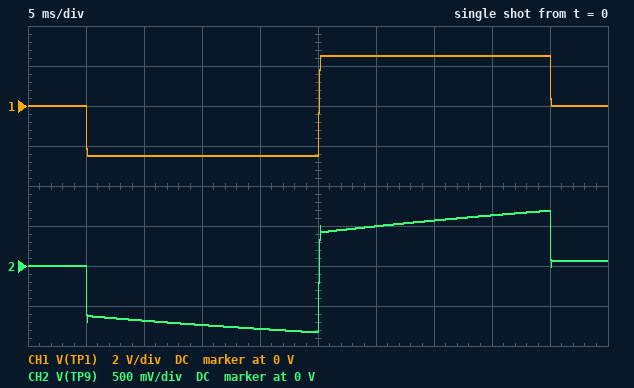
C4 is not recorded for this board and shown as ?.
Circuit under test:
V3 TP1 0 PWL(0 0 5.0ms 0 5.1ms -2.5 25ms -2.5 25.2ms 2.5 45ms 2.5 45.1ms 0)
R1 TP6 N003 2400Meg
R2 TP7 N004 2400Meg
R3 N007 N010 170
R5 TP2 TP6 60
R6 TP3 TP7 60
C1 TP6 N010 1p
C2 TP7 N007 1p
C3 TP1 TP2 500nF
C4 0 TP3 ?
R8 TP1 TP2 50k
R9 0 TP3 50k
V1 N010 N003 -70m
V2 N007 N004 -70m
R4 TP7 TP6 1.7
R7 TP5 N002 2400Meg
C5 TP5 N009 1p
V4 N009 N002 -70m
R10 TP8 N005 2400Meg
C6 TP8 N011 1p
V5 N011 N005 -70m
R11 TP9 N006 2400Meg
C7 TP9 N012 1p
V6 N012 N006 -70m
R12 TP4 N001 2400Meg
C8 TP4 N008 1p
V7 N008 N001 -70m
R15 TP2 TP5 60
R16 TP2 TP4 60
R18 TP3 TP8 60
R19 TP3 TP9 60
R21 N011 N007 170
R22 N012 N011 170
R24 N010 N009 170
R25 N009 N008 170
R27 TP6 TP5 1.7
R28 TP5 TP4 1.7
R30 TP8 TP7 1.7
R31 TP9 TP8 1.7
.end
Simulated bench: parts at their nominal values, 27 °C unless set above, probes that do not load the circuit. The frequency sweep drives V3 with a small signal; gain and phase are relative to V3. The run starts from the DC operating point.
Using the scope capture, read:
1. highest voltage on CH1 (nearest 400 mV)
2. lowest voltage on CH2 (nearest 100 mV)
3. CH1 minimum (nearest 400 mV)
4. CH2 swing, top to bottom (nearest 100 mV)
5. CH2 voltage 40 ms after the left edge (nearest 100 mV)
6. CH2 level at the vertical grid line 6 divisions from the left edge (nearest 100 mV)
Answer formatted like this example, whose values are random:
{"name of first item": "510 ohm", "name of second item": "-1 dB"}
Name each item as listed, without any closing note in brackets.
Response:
{"highest voltage on CH1": "2.4 V", "lowest voltage on CH2": "-800 mV", "CH1 minimum": "-2.4 V", "CH2 swing, top to bottom": "1.5 V", "CH2 voltage 40 ms after the left edge": "600 mV", "CH2 level at the vertical grid line 6 divisions from the left edge": "500 mV"}
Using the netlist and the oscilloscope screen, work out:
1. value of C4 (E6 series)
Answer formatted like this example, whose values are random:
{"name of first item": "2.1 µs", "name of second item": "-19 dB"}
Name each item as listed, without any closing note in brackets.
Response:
{"value of C4": "1.5 µF"}
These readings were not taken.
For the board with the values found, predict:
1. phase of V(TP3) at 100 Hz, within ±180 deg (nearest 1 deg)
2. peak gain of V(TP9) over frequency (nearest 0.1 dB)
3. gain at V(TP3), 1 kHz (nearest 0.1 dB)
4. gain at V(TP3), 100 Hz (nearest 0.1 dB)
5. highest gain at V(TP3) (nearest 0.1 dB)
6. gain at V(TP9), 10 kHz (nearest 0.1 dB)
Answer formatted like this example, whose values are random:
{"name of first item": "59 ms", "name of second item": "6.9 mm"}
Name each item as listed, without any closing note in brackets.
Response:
{"phase of V(TP3) at 100 Hz, within ±180 deg": "-2 deg", "peak gain of V(TP9) over frequency": "-6.0 dB", "gain at V(TP3), 1 kHz": "-12.1 dB", "gain at V(TP3), 100 Hz": "-12.0 dB", "highest gain at V(TP3)": "-6.0 dB", "gain at V(TP9), 10 kHz": "-8.8 dB"}
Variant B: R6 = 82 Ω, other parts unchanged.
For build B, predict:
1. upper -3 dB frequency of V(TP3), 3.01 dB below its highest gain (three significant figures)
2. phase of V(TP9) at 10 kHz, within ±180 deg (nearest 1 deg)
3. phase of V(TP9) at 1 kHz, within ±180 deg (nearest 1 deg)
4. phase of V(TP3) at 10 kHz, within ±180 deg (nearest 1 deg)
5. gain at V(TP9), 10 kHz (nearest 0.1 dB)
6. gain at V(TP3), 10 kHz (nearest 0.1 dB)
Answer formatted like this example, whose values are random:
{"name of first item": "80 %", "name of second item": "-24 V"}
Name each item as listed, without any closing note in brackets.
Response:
{"upper -3 dB frequency of V(TP3), 3.01 dB below its highest gain": "4.50 Hz", "phase of V(TP9) at 10 kHz, within ±180 deg": "16 deg", "phase of V(TP9) at 1 kHz, within ±180 deg": "5 deg", "phase of V(TP3) at 10 kHz, within ±180 deg": "-47 deg", "gain at V(TP9), 10 kHz": "-8.4 dB", "gain at V(TP3), 10 kHz": "-15.4 dB"}
